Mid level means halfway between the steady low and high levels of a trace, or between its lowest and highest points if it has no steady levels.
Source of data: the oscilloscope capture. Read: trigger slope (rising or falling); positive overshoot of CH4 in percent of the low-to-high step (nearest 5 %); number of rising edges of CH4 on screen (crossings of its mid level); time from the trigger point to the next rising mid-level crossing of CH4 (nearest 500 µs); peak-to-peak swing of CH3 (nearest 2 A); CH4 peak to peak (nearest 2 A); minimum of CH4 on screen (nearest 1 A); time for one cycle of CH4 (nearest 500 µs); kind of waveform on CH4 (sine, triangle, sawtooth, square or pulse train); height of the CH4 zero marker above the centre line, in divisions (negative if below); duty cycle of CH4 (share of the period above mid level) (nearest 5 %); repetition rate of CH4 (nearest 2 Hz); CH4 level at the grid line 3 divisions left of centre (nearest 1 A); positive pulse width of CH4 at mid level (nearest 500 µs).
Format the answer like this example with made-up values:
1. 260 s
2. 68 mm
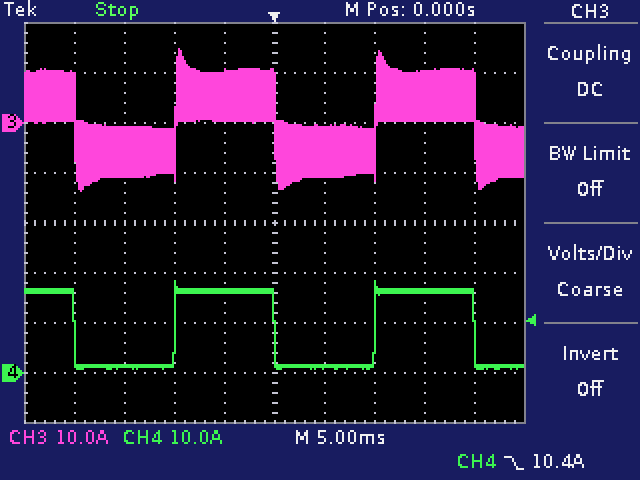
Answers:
1. falling
2. 15 %
3. 2
4. 10.0 ms
5. 28 A
6. 18 A
7. 1 A
8. 20.0 ms
9. square
10. -3.0 div
11. 50 %
12. 50 Hz
13. 1 A
14. 10.0 ms
